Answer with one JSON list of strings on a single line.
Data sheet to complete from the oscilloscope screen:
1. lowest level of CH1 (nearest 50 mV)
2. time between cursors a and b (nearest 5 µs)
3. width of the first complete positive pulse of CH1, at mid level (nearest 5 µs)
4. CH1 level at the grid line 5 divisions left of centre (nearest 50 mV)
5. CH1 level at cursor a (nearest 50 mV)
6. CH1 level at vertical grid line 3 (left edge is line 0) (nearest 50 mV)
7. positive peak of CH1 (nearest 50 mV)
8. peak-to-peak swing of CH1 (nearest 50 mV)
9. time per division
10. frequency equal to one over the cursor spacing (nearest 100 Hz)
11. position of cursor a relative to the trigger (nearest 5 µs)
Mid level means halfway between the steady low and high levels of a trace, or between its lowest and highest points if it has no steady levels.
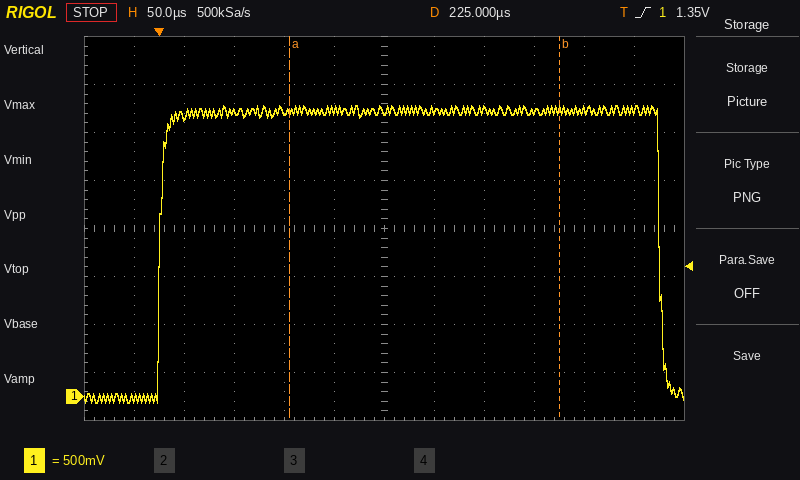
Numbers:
["-50 mV", "270 µs", "500 µs", "0 mV", "2.95 V", "2.95 V", "3.05 V", "3.10 V", "50 µs", "3.7 kHz", "+130 µs"]
